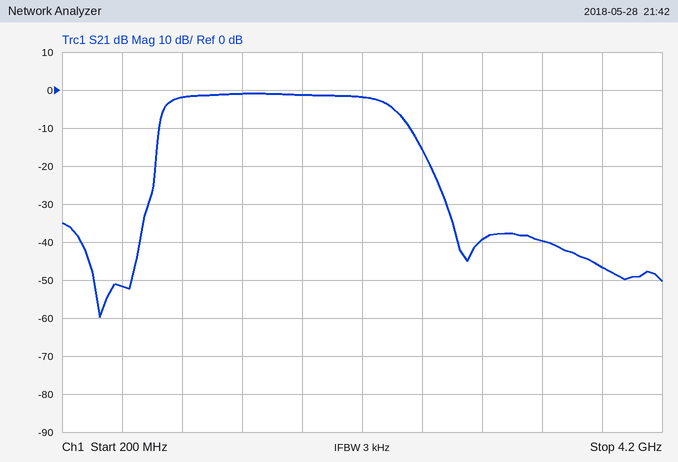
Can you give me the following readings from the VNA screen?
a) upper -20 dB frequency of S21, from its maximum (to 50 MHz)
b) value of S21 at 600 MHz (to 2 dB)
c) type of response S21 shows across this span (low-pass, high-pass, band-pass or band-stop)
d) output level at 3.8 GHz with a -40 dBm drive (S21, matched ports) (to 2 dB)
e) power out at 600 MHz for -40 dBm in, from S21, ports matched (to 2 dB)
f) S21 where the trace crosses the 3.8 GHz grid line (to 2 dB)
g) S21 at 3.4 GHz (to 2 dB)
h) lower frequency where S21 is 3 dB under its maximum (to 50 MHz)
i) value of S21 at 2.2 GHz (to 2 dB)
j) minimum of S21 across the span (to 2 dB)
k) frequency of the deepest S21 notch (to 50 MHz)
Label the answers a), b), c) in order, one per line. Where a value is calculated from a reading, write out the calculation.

a) 2.65 GHz
b) -52 dB
c) band-pass
d) -40 dBm + (-46 dB) = -86 dBm
e) -40 dBm + (-52 dB) = -92 dBm
f) -46 dB
g) -40 dB
h) 900 MHz
i) -2 dB
j) -60 dB
k) 450 MHz
